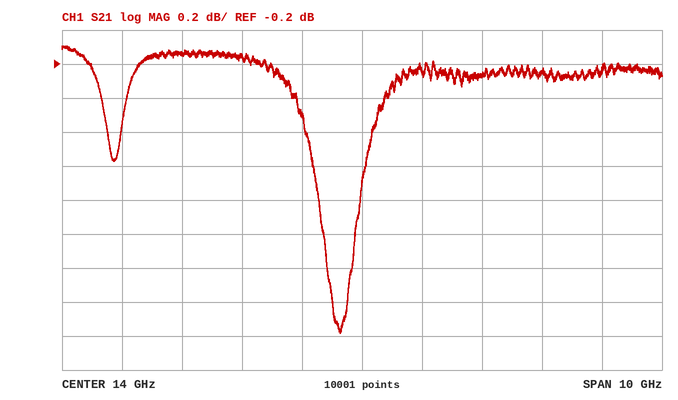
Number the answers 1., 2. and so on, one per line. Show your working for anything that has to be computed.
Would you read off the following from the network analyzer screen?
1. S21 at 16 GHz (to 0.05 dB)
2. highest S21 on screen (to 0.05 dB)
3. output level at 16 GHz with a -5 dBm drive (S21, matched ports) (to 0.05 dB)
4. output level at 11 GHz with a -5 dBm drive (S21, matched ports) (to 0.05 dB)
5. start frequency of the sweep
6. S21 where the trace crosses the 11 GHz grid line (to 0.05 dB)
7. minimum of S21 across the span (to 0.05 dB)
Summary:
1. -0.25 dB
2. -0.10 dB
3. -5 dBm + (-0.25 dB) = -5.25 dBm
4. -5 dBm + (-0.15 dB) = -5.15 dBm
5. 9 GHz
6. -0.15 dB
7. -1.80 dB
